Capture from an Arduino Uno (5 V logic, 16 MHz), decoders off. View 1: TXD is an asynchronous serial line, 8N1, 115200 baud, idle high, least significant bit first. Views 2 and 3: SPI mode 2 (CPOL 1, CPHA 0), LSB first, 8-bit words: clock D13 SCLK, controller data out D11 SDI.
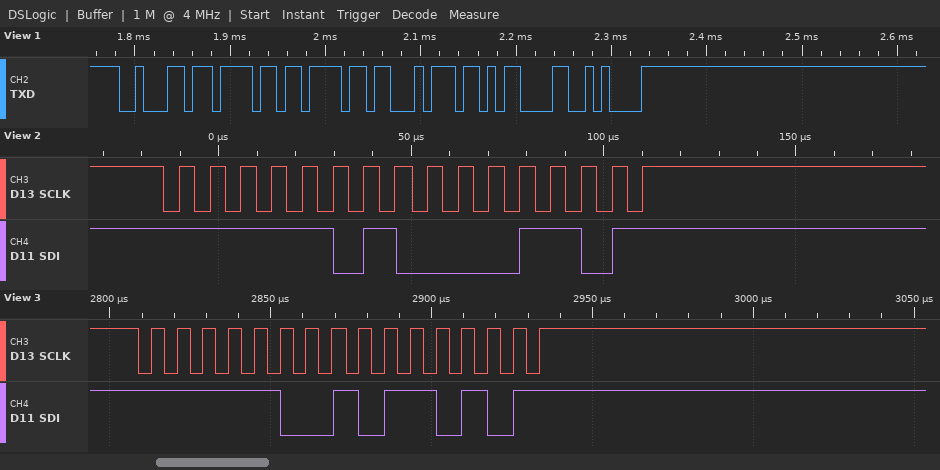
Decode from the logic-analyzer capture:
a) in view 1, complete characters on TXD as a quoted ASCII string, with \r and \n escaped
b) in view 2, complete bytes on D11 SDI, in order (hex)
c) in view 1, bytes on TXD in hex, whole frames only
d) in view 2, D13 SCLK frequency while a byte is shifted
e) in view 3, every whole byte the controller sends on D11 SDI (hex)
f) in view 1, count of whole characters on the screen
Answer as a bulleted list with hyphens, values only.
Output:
- "boot\r\n"
- BF B0
- 62 6F 6F 74 0D 0A
- 125 kHz
- 3F AD
- 6
